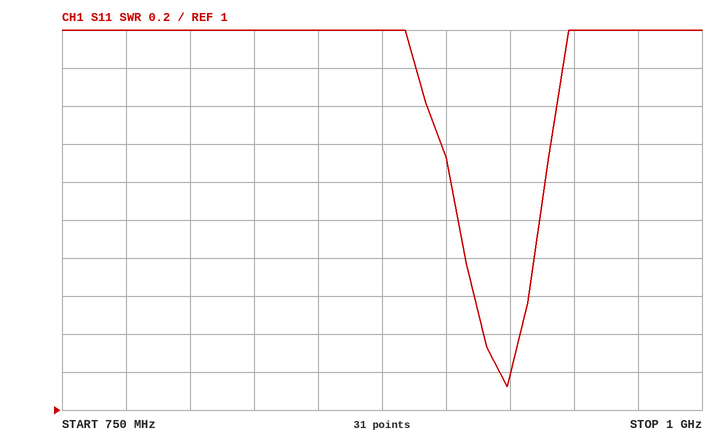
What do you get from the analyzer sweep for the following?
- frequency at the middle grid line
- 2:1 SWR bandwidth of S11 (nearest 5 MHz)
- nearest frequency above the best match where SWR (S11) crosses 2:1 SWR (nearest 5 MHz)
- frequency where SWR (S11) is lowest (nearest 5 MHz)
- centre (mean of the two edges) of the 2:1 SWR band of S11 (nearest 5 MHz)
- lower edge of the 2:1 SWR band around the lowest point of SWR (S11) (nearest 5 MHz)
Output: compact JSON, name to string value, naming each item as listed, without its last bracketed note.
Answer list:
{"frequency at the middle grid line": "875 MHz", "2:1 SWR bandwidth of S11": "30 MHz", "nearest frequency above the best match where SWR (S11) crosses 2:1 SWR": "935 MHz", "frequency where SWR (S11) is lowest": "925 MHz", "centre (mean of the two edges) of the 2:1 SWR band of S11": "920 MHz", "lower edge of the 2:1 SWR band around the lowest point of SWR (S11)": "905 MHz"}
